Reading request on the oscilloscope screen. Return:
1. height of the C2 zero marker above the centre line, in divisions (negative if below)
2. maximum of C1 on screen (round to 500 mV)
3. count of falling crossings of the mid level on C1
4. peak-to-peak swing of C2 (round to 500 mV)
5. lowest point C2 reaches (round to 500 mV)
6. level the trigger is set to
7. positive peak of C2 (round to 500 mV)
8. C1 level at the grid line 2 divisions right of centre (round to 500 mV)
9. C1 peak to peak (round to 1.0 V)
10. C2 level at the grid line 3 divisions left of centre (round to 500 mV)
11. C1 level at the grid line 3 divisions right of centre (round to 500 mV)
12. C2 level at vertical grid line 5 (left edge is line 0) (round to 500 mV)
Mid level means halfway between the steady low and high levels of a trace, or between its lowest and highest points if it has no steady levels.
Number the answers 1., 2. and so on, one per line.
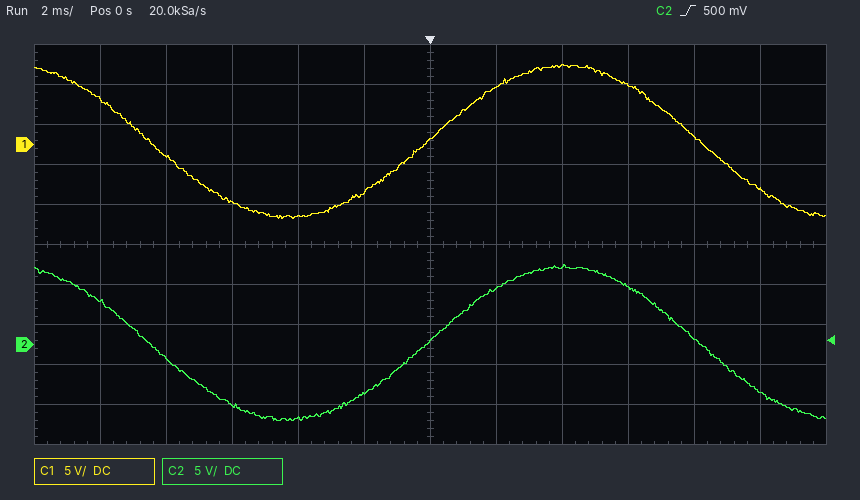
1. -2.5 div
2. 10.0 V
3. 2
4. 19.5 V
5. -9.5 V
6. 500 mV
7. 10.0 V
8. 10.0 V
9. 19.0 V
10. -7.5 V
11. 7.5 V
12. -6.0 V
